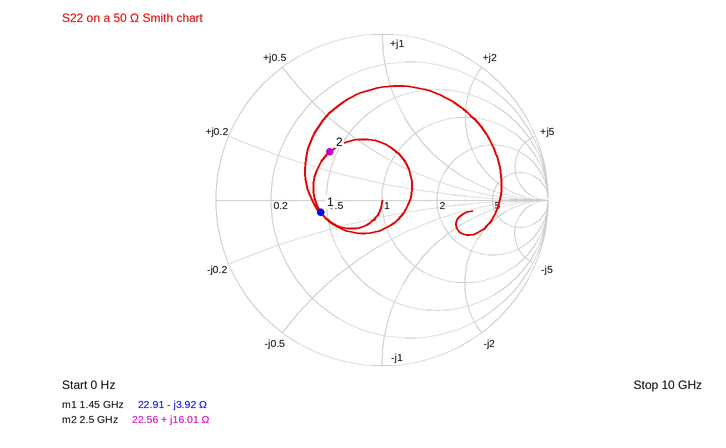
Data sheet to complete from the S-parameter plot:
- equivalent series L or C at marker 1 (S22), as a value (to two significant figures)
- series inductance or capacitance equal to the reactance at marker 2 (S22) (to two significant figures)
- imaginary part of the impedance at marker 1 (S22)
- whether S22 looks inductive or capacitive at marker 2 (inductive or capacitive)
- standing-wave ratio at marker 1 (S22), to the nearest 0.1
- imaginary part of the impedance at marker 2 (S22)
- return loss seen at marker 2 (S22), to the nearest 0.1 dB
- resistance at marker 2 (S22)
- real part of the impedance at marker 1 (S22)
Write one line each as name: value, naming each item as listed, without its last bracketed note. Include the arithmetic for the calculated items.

equivalent series L or C at marker 1 (S22), as a value: C = 1/(2π × 1.45 GHz × 3.92 Ω) ≈ 28 pF
series inductance or capacitance equal to the reactance at marker 2 (S22): L = 16.01 Ω/(2π × 2.5 GHz) ≈ 1.0 nH
imaginary part of the impedance at marker 1: -3.92 Ω
whether S22 looks inductive or capacitive at marker 2: inductive
standing-wave ratio at marker 1 (S22), to the nearest 0.1: 2.2
imaginary part of the impedance at marker 2: +16.01 Ω
return loss seen at marker 2 (S22), to the nearest 0.1 dB: 7.4 dB
resistance at marker 2: 22.56 Ω
real part of the impedance at marker 1: 22.91 Ω
